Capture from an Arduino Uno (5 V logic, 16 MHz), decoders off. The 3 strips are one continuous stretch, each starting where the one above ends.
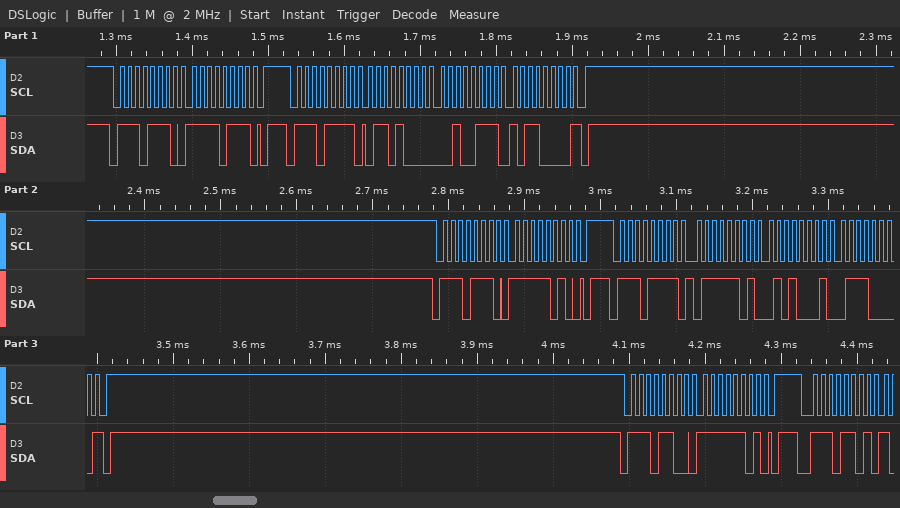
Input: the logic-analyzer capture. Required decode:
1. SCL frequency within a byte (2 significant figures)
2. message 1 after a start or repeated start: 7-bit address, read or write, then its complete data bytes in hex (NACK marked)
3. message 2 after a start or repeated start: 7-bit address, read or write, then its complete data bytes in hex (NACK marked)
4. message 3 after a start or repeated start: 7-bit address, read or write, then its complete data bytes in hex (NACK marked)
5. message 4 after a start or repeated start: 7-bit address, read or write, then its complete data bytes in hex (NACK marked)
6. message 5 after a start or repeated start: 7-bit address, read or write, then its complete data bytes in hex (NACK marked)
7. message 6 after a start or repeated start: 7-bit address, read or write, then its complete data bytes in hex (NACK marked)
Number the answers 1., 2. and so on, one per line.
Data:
1. 100 kHz
2. 0x77 write: F7
3. 0x77 read: 68 27 B0 NACK
4. 0x77 write: FA
5. 0x77 read: 7D 51 70 NACK
6. 0x76 write: FD
7. 0x76 read
